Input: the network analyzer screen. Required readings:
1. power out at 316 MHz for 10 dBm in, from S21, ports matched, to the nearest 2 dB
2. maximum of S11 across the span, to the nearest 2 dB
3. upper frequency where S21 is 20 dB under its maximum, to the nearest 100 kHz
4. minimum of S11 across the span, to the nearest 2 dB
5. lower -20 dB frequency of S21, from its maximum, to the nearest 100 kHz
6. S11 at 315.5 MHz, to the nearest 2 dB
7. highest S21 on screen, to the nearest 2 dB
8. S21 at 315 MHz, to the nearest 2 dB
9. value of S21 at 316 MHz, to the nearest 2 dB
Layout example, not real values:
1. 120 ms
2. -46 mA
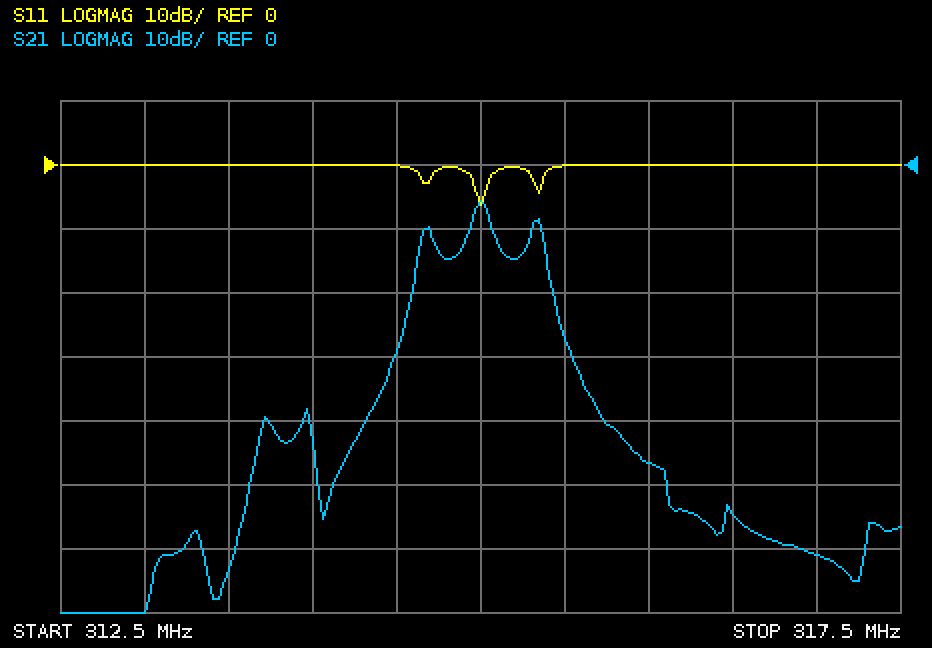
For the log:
1. -36 dBm
2. 0 dB
3. 315.5 MHz
4. -6 dB
5. 314.5 MHz
6. 0 dB
7. -6 dB
8. -6 dB
9. -46 dB
